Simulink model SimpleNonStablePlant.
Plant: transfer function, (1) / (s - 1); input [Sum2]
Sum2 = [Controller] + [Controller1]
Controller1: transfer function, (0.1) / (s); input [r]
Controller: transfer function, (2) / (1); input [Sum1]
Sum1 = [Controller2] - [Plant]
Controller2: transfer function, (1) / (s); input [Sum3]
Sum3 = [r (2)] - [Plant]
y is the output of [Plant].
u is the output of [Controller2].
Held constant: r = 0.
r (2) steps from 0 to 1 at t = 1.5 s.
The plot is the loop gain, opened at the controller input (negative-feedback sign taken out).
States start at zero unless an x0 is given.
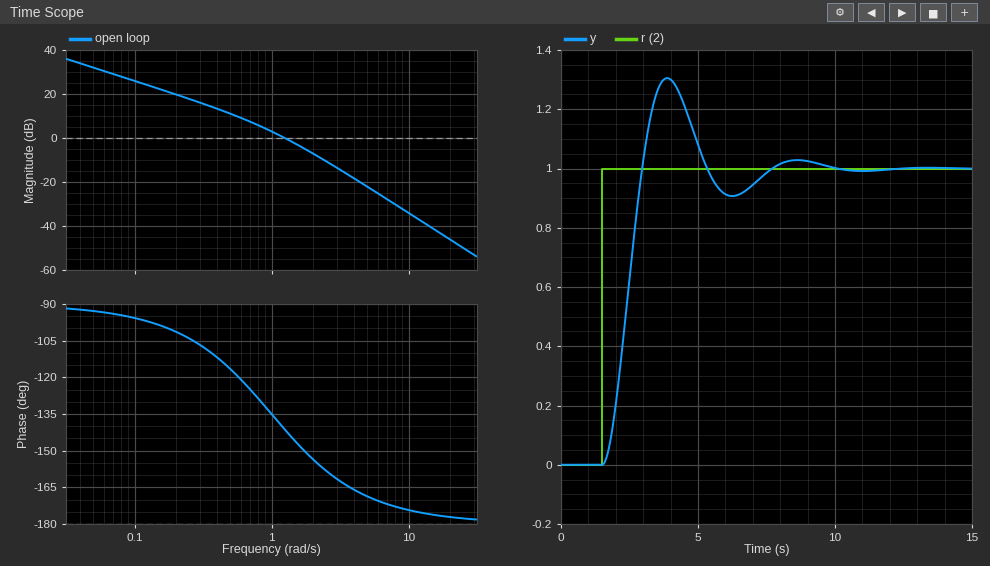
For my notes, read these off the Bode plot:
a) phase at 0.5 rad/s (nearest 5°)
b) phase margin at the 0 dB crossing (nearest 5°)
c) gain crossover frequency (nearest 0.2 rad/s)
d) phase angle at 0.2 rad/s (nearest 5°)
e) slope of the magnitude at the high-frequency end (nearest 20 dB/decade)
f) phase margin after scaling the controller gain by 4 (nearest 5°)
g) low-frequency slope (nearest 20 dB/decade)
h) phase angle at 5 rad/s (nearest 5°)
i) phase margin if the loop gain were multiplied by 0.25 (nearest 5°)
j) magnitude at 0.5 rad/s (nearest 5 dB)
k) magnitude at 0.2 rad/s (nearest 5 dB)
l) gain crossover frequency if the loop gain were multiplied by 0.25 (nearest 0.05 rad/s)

-115°
40°
1.2 rad/s
-100°
-40 dB/decade
20°
-20 dB/decade
-170°
65°
10 dB
20 dB
0.45 rad/s
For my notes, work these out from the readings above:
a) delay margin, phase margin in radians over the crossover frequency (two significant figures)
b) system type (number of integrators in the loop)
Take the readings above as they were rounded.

0.58 s
1
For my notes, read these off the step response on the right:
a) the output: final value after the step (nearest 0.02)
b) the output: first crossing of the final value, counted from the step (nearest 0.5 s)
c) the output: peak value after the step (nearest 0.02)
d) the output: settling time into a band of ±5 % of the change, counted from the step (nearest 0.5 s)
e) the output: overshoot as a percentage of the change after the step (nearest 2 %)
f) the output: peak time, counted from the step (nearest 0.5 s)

1.00
1.5 s
1.30
5.5 s
30 %
2.5 s
